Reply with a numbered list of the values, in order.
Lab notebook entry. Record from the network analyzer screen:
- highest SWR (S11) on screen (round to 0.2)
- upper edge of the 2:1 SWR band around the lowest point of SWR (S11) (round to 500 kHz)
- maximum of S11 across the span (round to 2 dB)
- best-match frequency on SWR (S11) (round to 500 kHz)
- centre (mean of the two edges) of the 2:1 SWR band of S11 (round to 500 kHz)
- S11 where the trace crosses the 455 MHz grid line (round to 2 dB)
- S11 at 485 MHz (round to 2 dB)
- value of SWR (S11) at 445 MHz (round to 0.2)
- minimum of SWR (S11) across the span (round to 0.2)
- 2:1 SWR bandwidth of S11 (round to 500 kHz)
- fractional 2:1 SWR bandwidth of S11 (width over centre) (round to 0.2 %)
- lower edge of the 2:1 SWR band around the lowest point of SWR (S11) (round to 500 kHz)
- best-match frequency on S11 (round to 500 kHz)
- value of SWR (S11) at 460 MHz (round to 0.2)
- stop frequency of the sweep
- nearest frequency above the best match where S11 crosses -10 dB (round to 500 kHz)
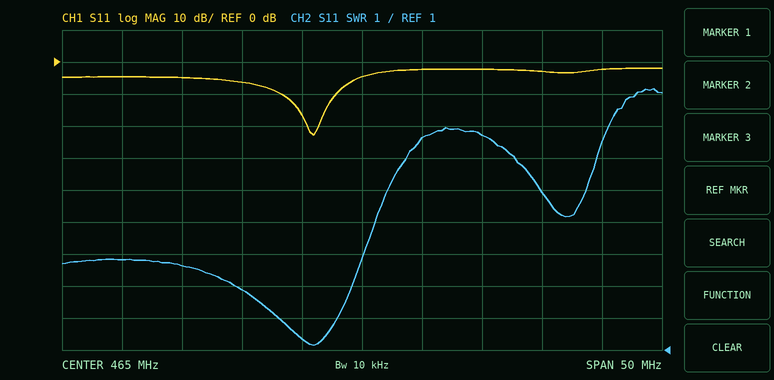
1. 9.2
2. 463.0 MHz
3. -2 dB
4. 461.0 MHz
5. 460.5 MHz
6. -6 dB
7. -2 dB
8. 3.8
9. 1.2
10. 5.0 MHz
11. 1.0 %
12. 458.0 MHz
13. 461.0 MHz
14. 1.4
15. 490 MHz
16. 463.0 MHz
